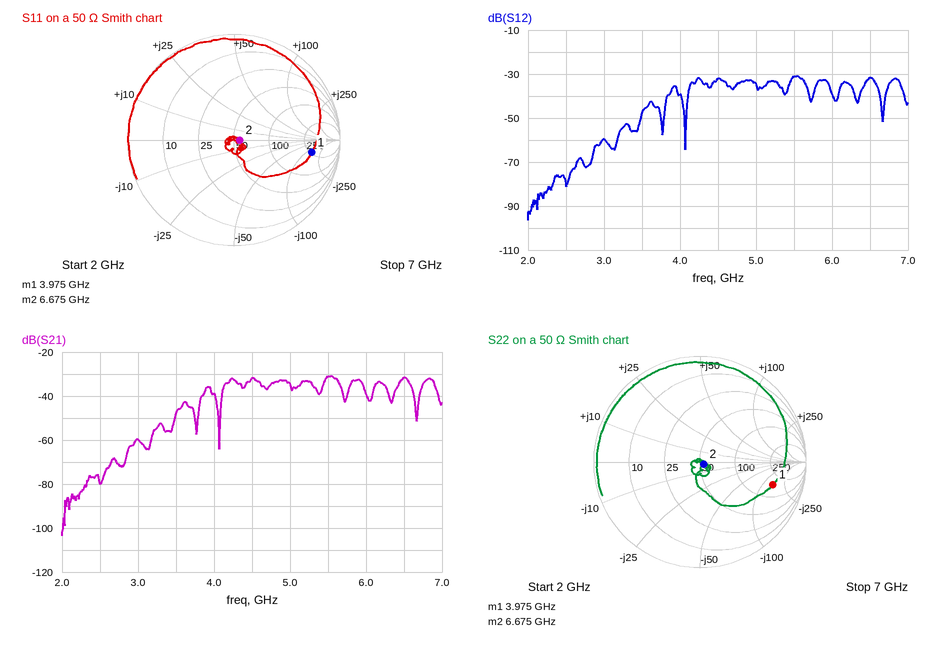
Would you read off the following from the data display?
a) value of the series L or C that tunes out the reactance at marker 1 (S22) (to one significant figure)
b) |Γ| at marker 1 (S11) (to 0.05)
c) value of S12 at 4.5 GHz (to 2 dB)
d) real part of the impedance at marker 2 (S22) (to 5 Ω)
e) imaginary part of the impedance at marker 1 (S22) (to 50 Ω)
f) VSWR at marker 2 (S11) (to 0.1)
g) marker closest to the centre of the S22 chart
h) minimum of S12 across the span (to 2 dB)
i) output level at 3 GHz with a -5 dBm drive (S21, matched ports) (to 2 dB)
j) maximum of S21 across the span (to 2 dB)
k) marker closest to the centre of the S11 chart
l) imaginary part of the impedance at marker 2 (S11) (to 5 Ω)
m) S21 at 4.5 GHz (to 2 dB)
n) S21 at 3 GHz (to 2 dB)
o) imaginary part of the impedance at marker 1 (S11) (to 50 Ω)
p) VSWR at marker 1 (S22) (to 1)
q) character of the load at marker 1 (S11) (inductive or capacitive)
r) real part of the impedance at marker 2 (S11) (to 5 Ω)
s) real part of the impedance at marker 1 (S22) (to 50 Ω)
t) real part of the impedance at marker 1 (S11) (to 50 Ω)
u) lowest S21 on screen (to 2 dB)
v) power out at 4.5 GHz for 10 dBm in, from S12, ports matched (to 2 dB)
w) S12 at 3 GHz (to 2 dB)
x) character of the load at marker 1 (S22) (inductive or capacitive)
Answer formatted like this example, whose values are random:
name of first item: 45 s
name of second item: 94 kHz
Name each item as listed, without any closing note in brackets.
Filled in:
value of the series L or C that tunes out the reactance at marker 1 (S22): 6 nH
|Γ| at marker 1 (S11): 0.75
value of S12 at 4.5 GHz: -32 dB
real part of the impedance at marker 2 (S22): 55 Ω
imaginary part of the impedance at marker 1 (S22): -150 Ω
VSWR at marker 2 (S11): 1.1
marker closest to the centre of the S22 chart: marker 2
minimum of S12 across the span: -96 dB
output level at 3 GHz with a -5 dBm drive (S21, matched ports): -64 dBm
maximum of S21 across the span: -30 dB
marker closest to the centre of the S11 chart: marker 2
imaginary part of the impedance at marker 2 (S11): 0 Ω
S21 at 4.5 GHz: -32 dB
S21 at 3 GHz: -60 dB
imaginary part of the impedance at marker 1 (S11): -150 Ω
VSWR at marker 1 (S22): 6
character of the load at marker 1 (S11): capacitive
real part of the impedance at marker 2 (S11): 55 Ω
real part of the impedance at marker 1 (S22): 150 Ω
real part of the impedance at marker 1 (S11): 250 Ω
lowest S21 on screen: -104 dB
power out at 4.5 GHz for 10 dBm in, from S12, ports matched: -22 dBm
S12 at 3 GHz: -60 dB
character of the load at marker 1 (S22): capacitive
